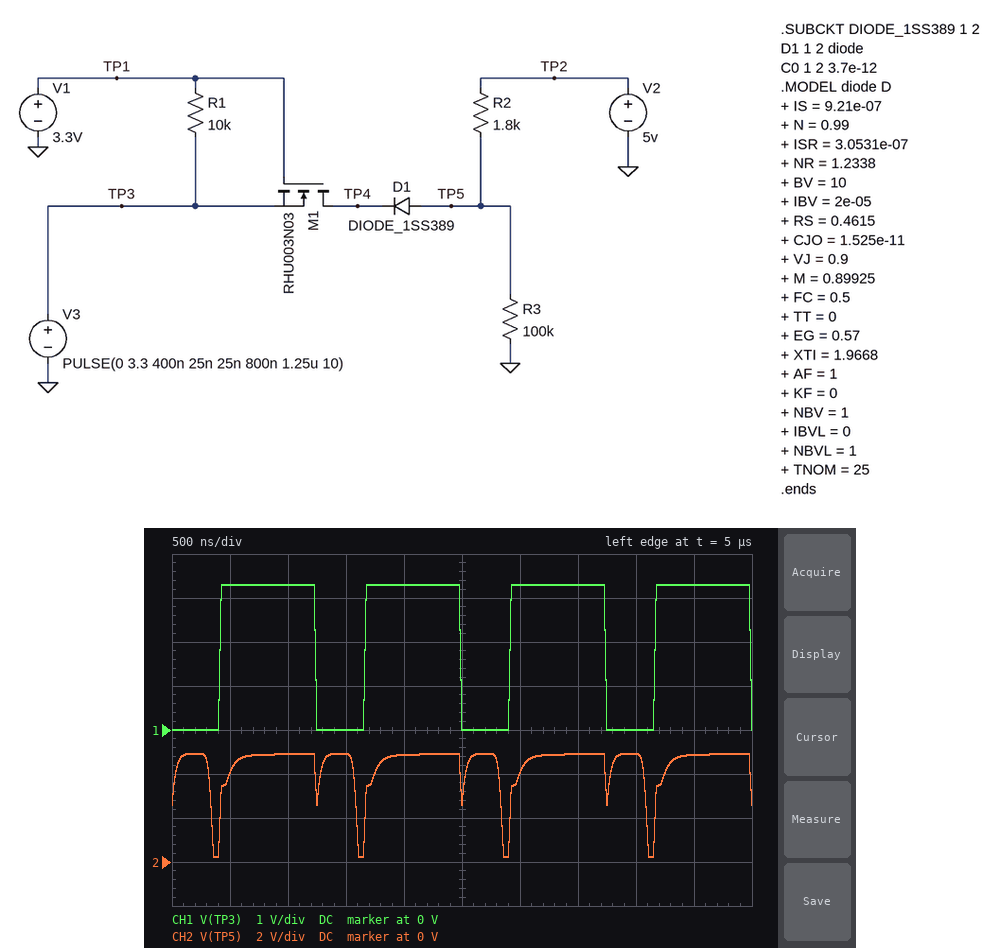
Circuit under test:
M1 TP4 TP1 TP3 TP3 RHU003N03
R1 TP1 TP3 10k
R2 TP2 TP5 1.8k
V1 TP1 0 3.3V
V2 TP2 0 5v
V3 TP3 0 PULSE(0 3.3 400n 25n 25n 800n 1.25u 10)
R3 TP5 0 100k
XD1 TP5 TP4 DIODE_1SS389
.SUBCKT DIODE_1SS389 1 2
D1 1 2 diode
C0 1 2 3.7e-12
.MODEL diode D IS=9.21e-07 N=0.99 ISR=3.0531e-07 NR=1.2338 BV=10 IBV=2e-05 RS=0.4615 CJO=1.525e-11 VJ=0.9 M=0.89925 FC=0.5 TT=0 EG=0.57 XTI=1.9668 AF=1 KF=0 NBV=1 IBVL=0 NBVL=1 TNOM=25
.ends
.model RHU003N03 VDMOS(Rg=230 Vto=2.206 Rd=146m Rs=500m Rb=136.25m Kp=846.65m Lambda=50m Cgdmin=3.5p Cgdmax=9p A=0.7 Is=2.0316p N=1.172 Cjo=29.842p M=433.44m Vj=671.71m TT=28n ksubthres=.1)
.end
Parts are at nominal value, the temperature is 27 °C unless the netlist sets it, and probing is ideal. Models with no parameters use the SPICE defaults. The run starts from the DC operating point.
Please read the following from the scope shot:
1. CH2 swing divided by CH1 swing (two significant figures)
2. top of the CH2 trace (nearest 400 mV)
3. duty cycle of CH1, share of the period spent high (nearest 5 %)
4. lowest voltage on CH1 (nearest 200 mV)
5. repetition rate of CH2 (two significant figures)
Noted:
1.4
4.8 V
65 %
0 V
800 kHz
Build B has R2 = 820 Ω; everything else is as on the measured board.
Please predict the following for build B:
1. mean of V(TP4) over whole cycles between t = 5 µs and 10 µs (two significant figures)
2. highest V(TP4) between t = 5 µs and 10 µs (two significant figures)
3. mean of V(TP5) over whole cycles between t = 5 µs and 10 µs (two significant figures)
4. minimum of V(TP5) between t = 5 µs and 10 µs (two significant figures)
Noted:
4.5 V
5.0 V
4.6 V
260 mV
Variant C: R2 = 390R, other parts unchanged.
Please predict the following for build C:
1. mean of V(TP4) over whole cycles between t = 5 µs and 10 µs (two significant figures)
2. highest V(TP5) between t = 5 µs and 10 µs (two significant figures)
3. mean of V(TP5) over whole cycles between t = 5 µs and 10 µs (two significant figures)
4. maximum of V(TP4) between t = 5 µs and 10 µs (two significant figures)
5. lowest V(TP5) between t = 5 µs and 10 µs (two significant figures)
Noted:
4.6 V
5.0 V
4.7 V
5.1 V
330 mV
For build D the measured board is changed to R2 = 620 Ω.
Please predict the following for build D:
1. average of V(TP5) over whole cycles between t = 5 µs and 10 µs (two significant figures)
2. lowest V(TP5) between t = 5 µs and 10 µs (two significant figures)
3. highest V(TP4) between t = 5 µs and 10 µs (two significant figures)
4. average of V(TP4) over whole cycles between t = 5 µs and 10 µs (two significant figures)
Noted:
4.6 V
280 mV
5.0 V
4.5 V
